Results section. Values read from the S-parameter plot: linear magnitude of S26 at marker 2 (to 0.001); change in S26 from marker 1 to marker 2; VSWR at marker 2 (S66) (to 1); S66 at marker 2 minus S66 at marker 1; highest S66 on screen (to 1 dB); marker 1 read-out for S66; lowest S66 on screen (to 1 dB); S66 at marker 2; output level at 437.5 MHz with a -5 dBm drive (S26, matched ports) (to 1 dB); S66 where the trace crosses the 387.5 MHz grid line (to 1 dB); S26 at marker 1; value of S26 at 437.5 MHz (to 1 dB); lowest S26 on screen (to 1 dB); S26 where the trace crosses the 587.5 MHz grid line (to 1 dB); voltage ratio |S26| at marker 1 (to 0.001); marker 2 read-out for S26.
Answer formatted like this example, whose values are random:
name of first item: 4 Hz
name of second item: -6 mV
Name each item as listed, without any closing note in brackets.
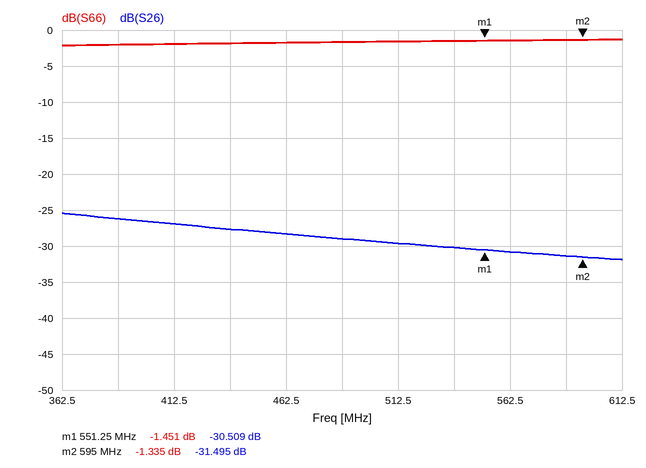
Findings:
linear magnitude of S26 at marker 2: 0.027
change in S26 from marker 1 to marker 2: -0.986 dB
VSWR at marker 2 (S66): 13
S66 at marker 2 minus S66 at marker 1: 0.116 dB
highest S66 on screen: -1 dB
marker 1 read-out for S66: -1.451 dB
lowest S66 on screen: -2 dB
S66 at marker 2: -1.335 dB
output level at 437.5 MHz with a -5 dBm drive (S26, matched ports): -33 dBm
S66 where the trace crosses the 387.5 MHz grid line: -2 dB
S26 at marker 1: -30.509 dB
value of S26 at 437.5 MHz: -28 dB
lowest S26 on screen: -32 dB
S26 where the trace crosses the 587.5 MHz grid line: -31 dB
voltage ratio |S26| at marker 1: 0.030
marker 2 read-out for S26: -31.495 dB
